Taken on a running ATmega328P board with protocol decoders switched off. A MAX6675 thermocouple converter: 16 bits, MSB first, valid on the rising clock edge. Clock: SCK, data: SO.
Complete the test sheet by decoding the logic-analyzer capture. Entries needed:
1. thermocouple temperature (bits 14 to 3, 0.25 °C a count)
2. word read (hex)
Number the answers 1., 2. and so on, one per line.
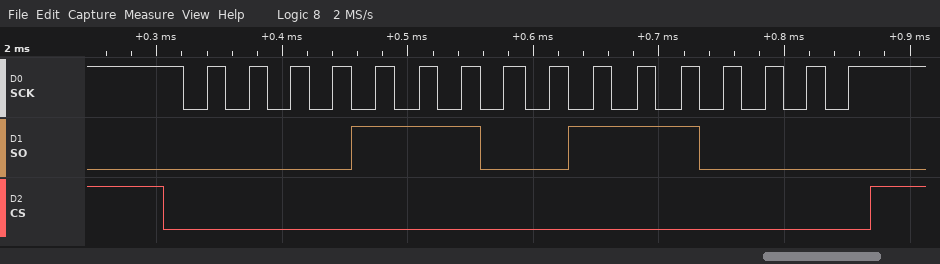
1. 115.50 °C
2. 0x0E70
